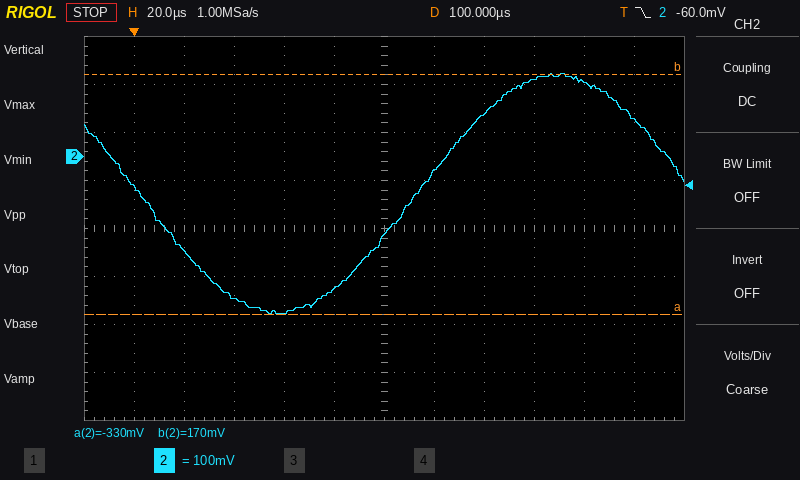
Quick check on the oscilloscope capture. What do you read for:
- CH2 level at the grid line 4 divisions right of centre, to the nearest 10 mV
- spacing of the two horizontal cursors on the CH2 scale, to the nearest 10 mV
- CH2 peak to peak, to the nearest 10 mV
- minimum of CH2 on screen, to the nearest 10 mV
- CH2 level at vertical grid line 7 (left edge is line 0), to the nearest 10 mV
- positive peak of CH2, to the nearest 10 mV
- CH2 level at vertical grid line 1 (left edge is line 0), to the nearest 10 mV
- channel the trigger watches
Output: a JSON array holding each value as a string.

["160 mV", "500 mV", "500 mV", "-330 mV", "-30 mV", "170 mV", "-60 mV", "CH2"]
